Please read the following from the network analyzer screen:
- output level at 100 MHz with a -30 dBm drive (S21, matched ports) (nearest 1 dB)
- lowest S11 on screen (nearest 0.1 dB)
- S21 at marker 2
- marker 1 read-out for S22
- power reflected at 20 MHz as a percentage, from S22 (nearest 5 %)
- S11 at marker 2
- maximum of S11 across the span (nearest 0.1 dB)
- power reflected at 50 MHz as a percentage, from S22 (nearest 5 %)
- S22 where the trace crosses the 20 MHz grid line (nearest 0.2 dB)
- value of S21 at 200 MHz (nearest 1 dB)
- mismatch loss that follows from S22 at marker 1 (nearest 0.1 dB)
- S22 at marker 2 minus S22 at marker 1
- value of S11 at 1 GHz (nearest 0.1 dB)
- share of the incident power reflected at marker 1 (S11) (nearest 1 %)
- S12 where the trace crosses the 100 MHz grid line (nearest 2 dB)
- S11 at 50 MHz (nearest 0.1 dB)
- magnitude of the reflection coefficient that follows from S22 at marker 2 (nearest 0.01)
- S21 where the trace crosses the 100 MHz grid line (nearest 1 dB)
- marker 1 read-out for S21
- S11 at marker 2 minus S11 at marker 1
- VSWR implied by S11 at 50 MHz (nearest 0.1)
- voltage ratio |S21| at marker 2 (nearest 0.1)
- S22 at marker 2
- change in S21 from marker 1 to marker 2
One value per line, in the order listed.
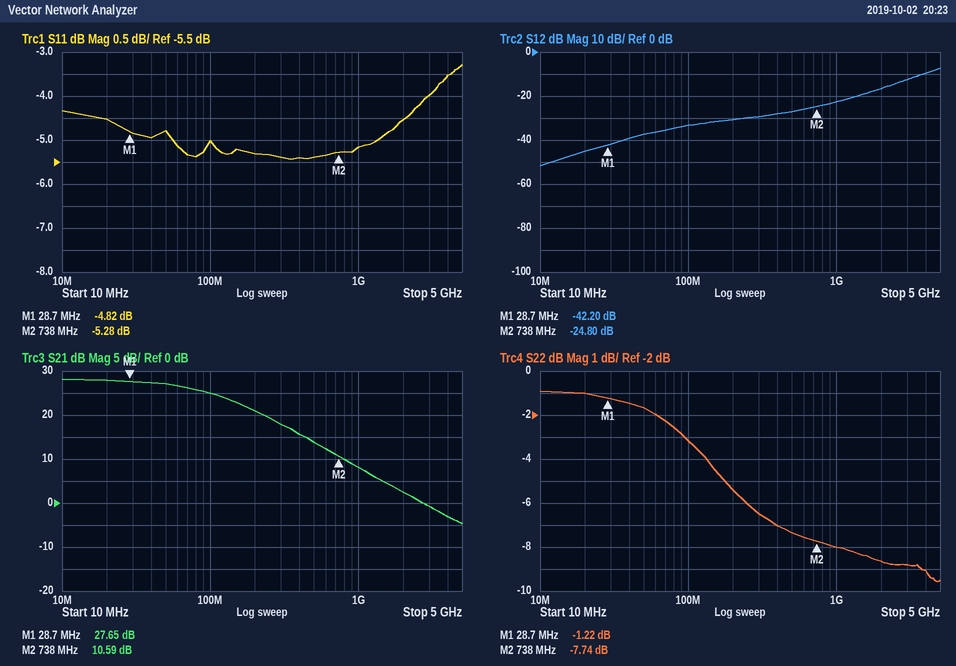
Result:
-5 dBm
-5.4 dB
10.59 dB
-1.22 dB
80 %
-5.28 dB
-3.3 dB
70 %
-1.0 dB
21 dB
6.1 dB
-6.52 dB
-5.2 dB
33 %
-34 dB
-4.8 dB
0.41
25 dB
27.65 dB
-0.46 dB
3.7
3.4
-7.74 dB
-17.06 dB
